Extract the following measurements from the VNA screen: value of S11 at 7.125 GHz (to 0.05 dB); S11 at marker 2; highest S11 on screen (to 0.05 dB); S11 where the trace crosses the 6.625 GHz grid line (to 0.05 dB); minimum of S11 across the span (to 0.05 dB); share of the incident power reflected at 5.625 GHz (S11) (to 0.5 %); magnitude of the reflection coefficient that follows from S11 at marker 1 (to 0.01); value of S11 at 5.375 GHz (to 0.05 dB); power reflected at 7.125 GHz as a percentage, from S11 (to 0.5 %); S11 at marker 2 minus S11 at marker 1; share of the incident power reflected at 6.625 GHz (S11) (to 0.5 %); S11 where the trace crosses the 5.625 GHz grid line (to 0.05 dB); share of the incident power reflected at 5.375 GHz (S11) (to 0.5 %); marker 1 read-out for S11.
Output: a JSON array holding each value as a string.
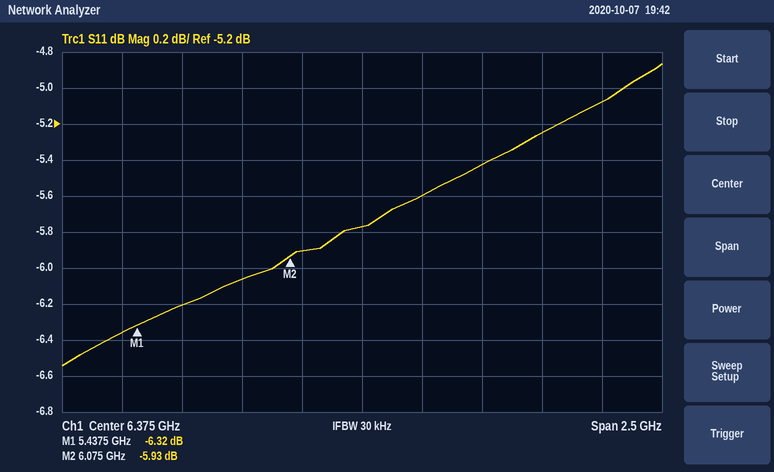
["-5.25 dB", "-5.93 dB", "-4.85 dB", "-5.60 dB", "-6.55 dB", "24.0 %", "0.48", "-6.35 dB", "30.0 %", "0.39 dB", "27.5 %", "-6.20 dB", "23.0 %", "-6.32 dB"]
